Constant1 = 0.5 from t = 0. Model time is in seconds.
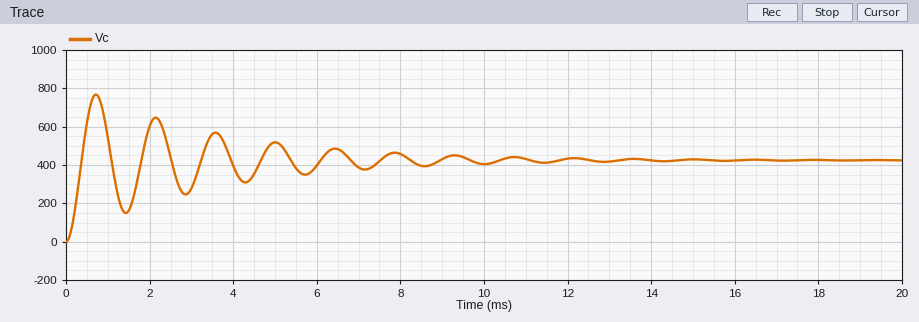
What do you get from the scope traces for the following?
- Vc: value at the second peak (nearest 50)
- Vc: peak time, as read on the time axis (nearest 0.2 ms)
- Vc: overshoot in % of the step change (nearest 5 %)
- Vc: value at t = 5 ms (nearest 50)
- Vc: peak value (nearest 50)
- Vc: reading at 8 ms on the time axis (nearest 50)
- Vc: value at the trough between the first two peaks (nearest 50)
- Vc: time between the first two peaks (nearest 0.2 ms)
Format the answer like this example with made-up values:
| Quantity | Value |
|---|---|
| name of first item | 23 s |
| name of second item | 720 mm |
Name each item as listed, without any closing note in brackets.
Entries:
| Quantity | Value |
|---|---|
| Vc: value at the second peak | 650 |
| Vc: peak time, as read on the time axis | 0.8 ms |
| Vc: overshoot in % of the step change | 80 % |
| Vc: value at t = 5 ms | 500 |
| Vc: peak value | 750 |
| Vc: reading at 8 ms on the time axis | 450 |
| Vc: value at the trough between the first two peaks | 150 |
| Vc: time between the first two peaks | 1.4 ms |
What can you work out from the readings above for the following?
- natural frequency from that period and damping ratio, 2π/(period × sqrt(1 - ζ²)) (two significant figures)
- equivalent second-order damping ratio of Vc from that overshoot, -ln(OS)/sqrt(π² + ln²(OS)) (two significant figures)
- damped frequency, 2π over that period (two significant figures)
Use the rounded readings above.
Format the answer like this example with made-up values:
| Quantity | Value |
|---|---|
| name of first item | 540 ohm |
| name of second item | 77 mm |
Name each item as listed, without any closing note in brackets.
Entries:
| Quantity | Value |
|---|---|
| natural frequency from that period and damping ratio, 2π/(period × sqrt(1 - ζ²)) | 4.5 rad/ms |
| equivalent second-order damping ratio of Vc from that overshoot, -ln(OS)/sqrt(π² + ln²(OS)) | 0.071 |
| damped frequency, 2π over that period | 4.5 rad/ms |
